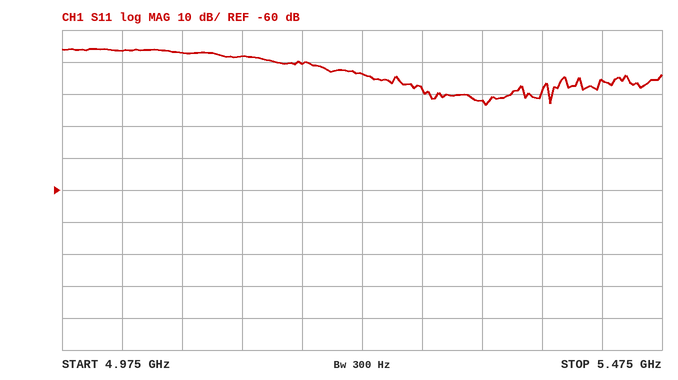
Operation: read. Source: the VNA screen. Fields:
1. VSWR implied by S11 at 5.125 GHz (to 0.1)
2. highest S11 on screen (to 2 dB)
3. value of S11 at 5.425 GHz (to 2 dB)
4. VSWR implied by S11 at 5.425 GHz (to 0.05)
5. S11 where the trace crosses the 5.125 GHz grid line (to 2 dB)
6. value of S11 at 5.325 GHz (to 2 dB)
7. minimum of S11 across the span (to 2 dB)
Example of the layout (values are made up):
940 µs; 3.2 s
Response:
1.3; -16 dB; -26 dB; 1.10; -18 dB; -32 dB; -34 dB
